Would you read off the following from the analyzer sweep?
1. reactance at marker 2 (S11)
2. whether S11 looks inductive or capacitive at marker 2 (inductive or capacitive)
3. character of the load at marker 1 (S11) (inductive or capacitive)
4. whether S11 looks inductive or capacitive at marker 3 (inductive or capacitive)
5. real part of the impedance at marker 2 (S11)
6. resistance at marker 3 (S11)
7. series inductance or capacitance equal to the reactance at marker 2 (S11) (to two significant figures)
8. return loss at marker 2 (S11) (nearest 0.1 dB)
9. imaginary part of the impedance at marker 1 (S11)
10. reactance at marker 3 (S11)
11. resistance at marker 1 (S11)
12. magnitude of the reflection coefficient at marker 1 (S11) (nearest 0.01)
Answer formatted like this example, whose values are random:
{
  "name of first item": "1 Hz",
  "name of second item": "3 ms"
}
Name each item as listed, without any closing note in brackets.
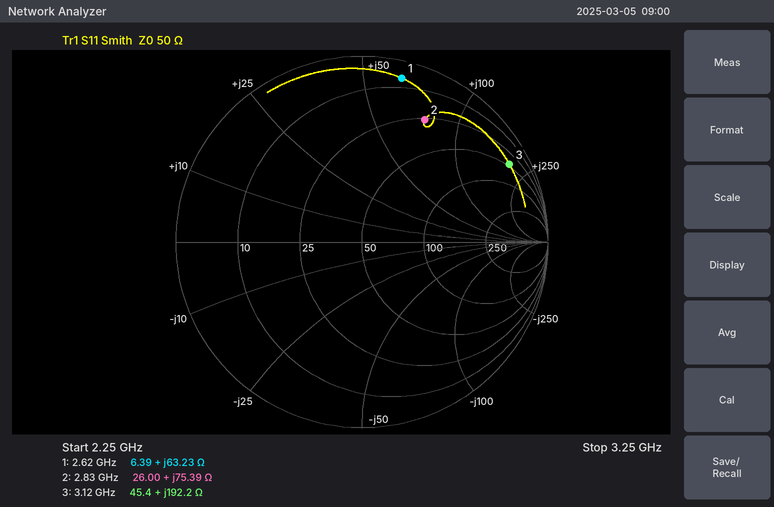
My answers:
{
  "reactance at marker 2": "+75.39 Ω",
  "whether S11 looks inductive or capacitive at marker 2": "inductive",
  "character of the load at marker 1 (S11)": "inductive",
  "whether S11 looks inductive or capacitive at marker 3": "inductive",
  "real part of the impedance at marker 2": "26.00 Ω",
  "resistance at marker 3": "45.4 Ω",
  "series inductance or capacitance equal to the reactance at marker 2 (S11)": "4.2 nH",
  "return loss at marker 2 (S11)": "2.6 dB",
  "imaginary part of the impedance at marker 1": "+63.23 Ω",
  "reactance at marker 3": "+192.2 Ω",
  "resistance at marker 1": "6.39 Ω",
  "magnitude of the reflection coefficient at marker 1 (S11)": "0.91"
}
